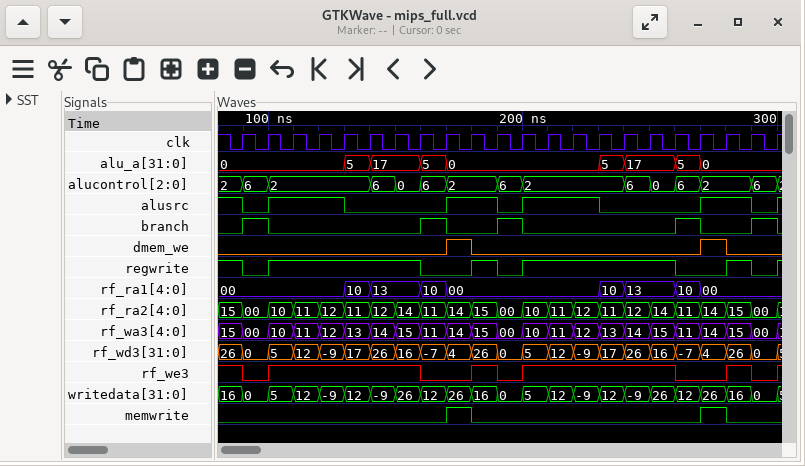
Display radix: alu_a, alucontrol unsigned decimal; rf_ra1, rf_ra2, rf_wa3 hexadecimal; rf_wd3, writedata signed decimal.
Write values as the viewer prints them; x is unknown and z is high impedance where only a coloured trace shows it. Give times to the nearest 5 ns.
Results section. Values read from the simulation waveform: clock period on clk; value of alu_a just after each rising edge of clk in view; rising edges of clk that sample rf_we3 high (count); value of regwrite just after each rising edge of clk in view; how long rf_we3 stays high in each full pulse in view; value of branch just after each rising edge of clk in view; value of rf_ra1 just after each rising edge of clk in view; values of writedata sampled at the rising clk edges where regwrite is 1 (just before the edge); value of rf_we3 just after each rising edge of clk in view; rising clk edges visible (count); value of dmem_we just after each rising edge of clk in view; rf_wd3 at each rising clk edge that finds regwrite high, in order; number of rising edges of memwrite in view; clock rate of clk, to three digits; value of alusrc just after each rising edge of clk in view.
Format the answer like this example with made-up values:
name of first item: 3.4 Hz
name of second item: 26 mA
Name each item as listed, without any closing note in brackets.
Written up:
clock period on clk: 10 ns
value of alu_a just after each rising edge of clk in view: 0, 0, 0, 0, 5, 17, 17, 5, 0, 0, 0, 0, 0, 0, 5, 17, 17, 5, 0, 0, 0, 0
rising edges of clk that sample rf_we3 high: 15
value of regwrite just after each rising edge of clk in view: 0 1 1 1 1 1 1 0 0 1 0 1 1 1 1 1 1 0 0 1 0 1
how long rf_we3 stays high in each full pulse in view: 60 ns, 10 ns, 60 ns, 10 ns
value of branch just after each rising edge of clk in view: 1 0 0 0 0 0 0 1 0 0 1 0 0 0 0 0 0 1 0 0 1 0
value of rf_ra1 just after each rising edge of clk in view: 00, 00, 00, 00, 10, 13, 13, 10, 00, 00, 00, 00, 00, 00, 10, 13, 13, 10, 00, 00, 00, 00
values of writedata sampled at the rising clk edges where regwrite is 1: 16, 5, 12, -9, 12, -9, 26, 16, 5, 12, -9, 12, -9, 26, 16
value of rf_we3 just after each rising edge of clk in view: 0 1 1 1 1 1 1 0 0 1 0 1 1 1 1 1 1 0 0 1 0 1
rising clk edges visible: 22
value of dmem_we just after each rising edge of clk in view: 0 0 0 0 0 0 0 0 1 0 0 0 0 0 0 0 0 0 1 0 0 0
rf_wd3 at each rising clk edge that finds regwrite high, in order: 26, 5, 12, -9, 17, 26, 16, 26, 5, 12, -9, 17, 26, 16, 26
number of rising edges of memwrite in view: 2
clock rate of clk, to three digits: 100 MHz
value of alusrc just after each rising edge of clk in view: 0 1 1 1 0 0 0 0 1 1 0 1 1 1 0 0 0 0 1 1 0 1
